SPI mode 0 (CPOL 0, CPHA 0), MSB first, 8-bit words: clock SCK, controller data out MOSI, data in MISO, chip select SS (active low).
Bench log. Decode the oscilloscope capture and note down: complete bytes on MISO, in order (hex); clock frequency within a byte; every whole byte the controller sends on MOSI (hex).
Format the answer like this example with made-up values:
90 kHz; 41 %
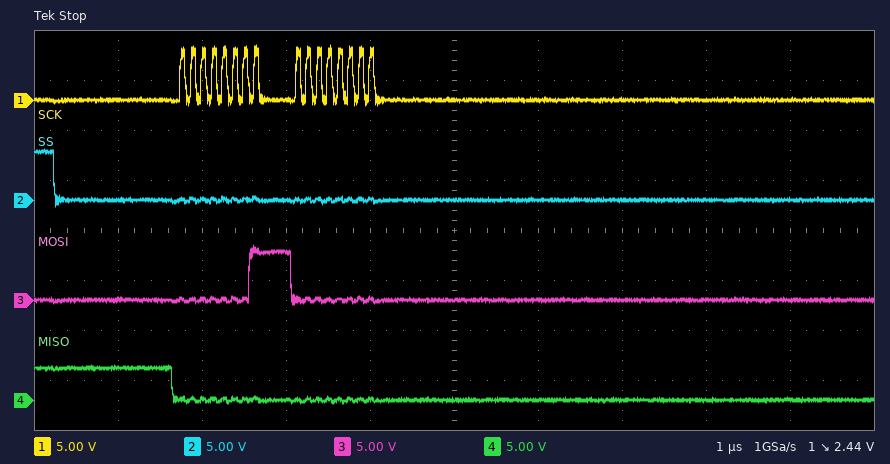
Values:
00 00; 8 MHz; 01 00
